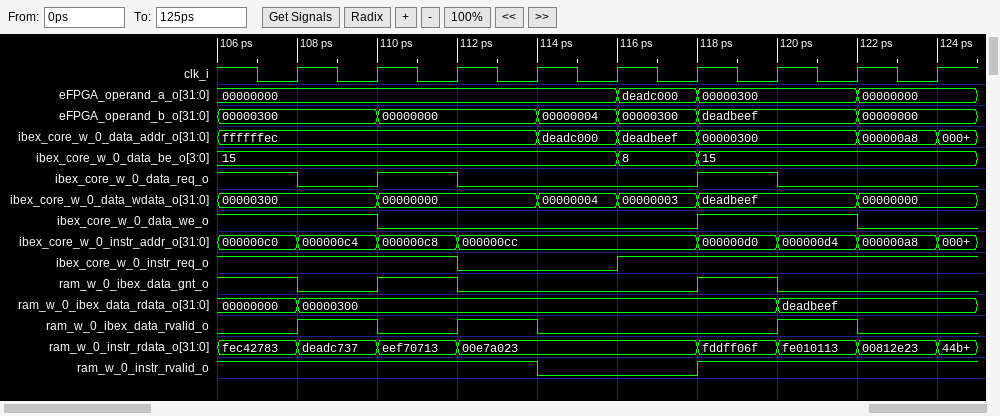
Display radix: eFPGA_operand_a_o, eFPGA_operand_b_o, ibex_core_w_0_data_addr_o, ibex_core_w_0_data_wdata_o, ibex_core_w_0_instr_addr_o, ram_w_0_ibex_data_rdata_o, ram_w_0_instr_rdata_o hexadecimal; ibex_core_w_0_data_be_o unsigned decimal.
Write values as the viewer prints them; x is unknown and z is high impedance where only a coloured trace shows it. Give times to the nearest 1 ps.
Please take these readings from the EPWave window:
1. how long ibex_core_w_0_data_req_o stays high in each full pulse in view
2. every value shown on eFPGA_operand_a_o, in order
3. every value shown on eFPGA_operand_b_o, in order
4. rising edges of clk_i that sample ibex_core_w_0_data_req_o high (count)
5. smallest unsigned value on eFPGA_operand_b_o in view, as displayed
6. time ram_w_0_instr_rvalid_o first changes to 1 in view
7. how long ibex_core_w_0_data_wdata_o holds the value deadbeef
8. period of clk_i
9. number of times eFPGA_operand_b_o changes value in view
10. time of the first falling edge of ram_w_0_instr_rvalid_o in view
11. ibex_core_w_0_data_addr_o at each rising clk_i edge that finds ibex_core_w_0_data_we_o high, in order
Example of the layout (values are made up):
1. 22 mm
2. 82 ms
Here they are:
1. 2 ps, 2 ps
2. 00000000, deadc000, 00000300, 00000000
3. 00000300, 00000000, 00000004, 00000300, deadbeef, 00000000
4. 3
5. 00000000
6. 118 ps
7. 4 ps
8. 2 ps
9. 5
10. 114 ps
11. ffffffec, ffffffec, 00000300, 00000300
